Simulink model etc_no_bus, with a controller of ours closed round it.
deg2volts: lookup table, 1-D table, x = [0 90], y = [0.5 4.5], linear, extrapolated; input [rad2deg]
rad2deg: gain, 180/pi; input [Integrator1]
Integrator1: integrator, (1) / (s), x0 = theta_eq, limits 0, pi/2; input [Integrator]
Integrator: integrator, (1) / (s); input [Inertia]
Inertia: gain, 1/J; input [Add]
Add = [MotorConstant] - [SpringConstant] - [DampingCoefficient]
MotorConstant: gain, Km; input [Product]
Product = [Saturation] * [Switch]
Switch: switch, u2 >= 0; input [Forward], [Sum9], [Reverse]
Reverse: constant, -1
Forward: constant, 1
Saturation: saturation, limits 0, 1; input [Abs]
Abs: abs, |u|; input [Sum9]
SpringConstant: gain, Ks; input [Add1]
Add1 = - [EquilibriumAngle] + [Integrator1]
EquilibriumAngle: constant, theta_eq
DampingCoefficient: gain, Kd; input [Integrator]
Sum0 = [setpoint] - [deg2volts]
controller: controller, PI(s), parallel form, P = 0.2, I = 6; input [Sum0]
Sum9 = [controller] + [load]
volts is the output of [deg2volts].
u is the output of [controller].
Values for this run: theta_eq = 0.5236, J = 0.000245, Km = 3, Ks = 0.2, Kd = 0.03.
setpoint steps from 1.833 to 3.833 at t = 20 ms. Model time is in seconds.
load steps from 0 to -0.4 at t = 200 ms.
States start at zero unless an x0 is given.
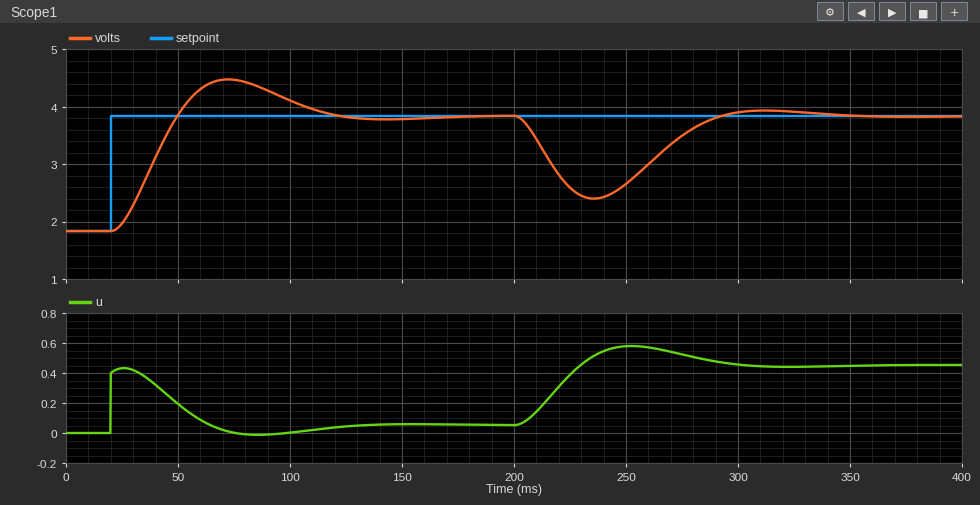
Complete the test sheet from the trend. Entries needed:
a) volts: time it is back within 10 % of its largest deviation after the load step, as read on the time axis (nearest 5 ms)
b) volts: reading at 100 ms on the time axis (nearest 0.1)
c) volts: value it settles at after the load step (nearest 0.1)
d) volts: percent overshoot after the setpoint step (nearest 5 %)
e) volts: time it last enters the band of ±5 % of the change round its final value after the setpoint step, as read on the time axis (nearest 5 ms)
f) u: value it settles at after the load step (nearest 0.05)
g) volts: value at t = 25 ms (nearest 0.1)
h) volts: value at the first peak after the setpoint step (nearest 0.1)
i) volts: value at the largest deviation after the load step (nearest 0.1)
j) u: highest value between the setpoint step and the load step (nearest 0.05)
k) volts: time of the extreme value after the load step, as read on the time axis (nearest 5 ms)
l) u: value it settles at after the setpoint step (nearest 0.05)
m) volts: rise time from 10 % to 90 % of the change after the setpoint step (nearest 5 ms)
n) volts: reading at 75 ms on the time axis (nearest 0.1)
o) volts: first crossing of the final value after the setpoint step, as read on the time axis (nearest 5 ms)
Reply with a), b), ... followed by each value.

a) 285 ms
b) 4.1
c) 3.8
d) 30 %
e) 110 ms
f) 0.45
g) 2.0
h) 4.5
i) 2.4
j) 0.45
k) 235 ms
l) 0.05
m) 20 ms
n) 4.5
o) 50 ms
